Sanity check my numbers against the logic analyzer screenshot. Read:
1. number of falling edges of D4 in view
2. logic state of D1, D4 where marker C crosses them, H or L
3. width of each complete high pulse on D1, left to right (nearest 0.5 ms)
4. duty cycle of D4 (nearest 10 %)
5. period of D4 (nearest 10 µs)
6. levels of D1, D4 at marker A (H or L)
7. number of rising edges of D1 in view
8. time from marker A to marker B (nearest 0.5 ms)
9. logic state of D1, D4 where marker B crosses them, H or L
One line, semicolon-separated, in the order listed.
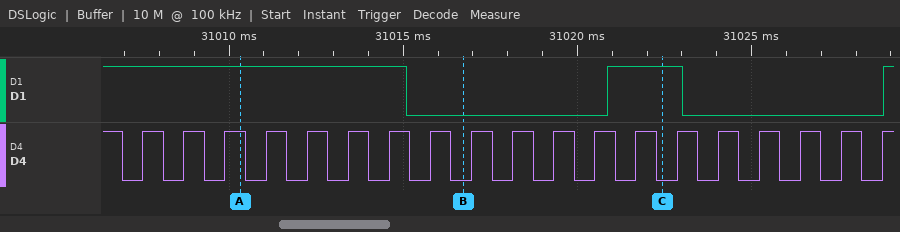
19; D1=H, D4=L; 2 ms; 50 %; 1180 µs; D1=H, D4=H; 2; 6.5 ms; D1=L, D4=L
